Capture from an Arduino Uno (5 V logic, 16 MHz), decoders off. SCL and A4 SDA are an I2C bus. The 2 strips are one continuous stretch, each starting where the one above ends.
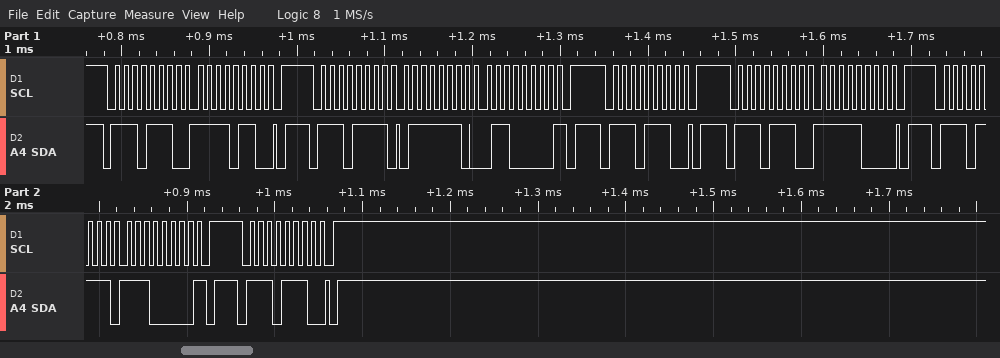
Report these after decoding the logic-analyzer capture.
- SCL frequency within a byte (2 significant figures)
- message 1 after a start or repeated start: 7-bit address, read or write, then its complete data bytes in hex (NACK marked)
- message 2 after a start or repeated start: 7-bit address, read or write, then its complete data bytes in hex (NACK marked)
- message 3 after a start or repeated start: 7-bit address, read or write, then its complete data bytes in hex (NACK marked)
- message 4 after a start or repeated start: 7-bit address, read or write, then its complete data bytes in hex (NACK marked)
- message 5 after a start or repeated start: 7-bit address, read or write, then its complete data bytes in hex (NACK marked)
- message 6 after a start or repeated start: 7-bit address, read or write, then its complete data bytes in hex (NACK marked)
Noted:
100 kHz
0x77 write: F6
0x77 read: 7E 60 NACK
0x77 write
0x77 write: F8
0x77 read: E0 NACK
0x77 write
